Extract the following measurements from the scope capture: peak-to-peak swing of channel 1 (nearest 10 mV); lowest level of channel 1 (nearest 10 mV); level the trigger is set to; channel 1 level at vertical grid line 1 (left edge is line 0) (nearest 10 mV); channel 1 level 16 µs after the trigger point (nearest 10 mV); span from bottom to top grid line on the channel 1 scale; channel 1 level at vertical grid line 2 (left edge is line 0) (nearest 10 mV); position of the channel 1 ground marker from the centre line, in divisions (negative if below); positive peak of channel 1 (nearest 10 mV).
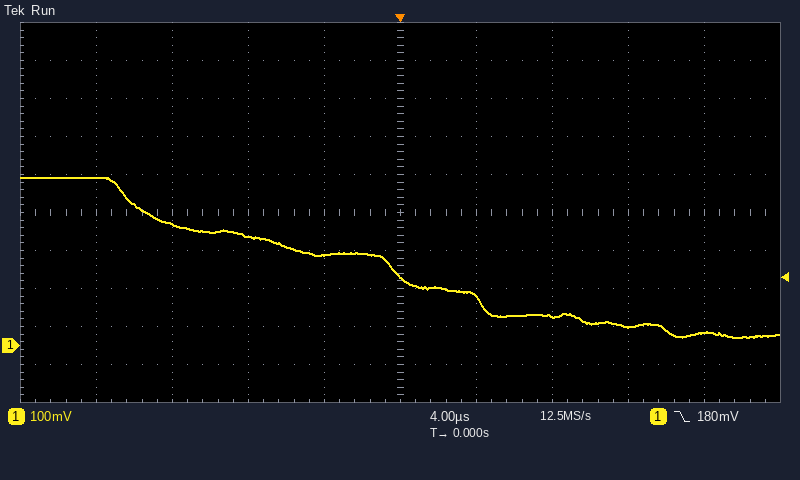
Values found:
420 mV
20 mV
180 mV
440 mV
30 mV
1 V
320 mV
-3.5 div
440 mV
